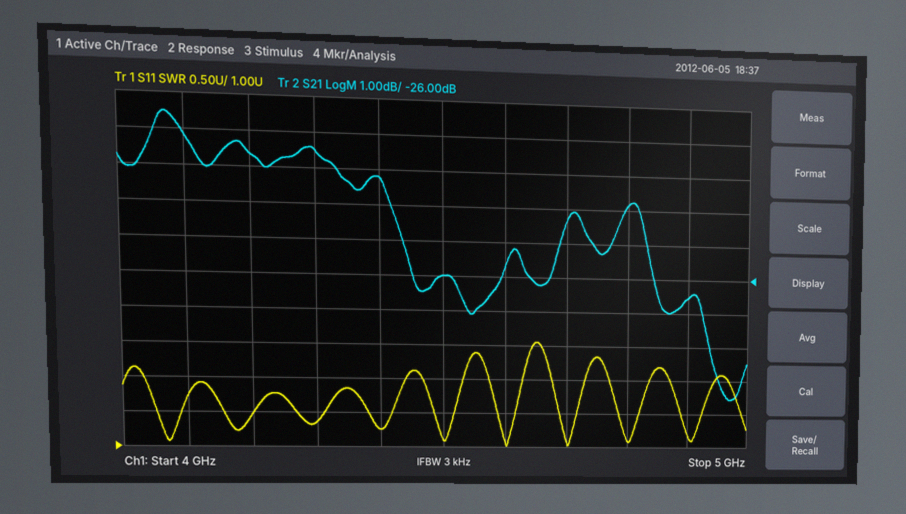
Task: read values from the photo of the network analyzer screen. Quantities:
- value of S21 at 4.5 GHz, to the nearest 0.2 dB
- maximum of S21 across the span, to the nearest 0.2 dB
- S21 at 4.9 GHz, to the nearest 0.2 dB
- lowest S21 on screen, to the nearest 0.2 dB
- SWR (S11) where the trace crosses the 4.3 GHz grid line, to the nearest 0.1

-26.0 dB
-21.6 dB
-26.6 dB
-29.6 dB
1.4
